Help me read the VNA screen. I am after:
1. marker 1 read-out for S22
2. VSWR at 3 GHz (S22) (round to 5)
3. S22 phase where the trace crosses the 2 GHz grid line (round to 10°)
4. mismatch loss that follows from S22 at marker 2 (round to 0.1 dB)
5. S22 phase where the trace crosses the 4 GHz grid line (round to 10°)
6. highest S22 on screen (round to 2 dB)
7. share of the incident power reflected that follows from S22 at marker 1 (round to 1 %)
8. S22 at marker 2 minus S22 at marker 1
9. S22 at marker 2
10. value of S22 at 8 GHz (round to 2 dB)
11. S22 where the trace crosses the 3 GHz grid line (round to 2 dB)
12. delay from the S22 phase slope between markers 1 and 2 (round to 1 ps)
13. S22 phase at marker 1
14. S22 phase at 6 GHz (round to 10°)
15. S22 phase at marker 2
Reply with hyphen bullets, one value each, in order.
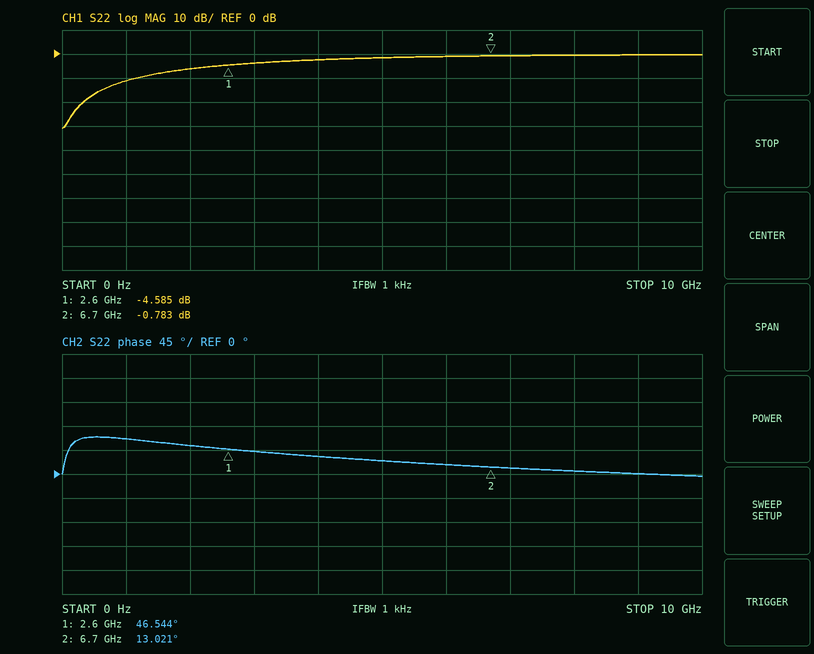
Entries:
- -4.585 dB
- 5
- 50°
- 7.8 dB
- 30°
- 0 dB
- 35 %
- 3.802 dB
- -0.783 dB
- 0 dB
- -4 dB
- 23 ps
- 46.544°
- 20°
- 13.021°
